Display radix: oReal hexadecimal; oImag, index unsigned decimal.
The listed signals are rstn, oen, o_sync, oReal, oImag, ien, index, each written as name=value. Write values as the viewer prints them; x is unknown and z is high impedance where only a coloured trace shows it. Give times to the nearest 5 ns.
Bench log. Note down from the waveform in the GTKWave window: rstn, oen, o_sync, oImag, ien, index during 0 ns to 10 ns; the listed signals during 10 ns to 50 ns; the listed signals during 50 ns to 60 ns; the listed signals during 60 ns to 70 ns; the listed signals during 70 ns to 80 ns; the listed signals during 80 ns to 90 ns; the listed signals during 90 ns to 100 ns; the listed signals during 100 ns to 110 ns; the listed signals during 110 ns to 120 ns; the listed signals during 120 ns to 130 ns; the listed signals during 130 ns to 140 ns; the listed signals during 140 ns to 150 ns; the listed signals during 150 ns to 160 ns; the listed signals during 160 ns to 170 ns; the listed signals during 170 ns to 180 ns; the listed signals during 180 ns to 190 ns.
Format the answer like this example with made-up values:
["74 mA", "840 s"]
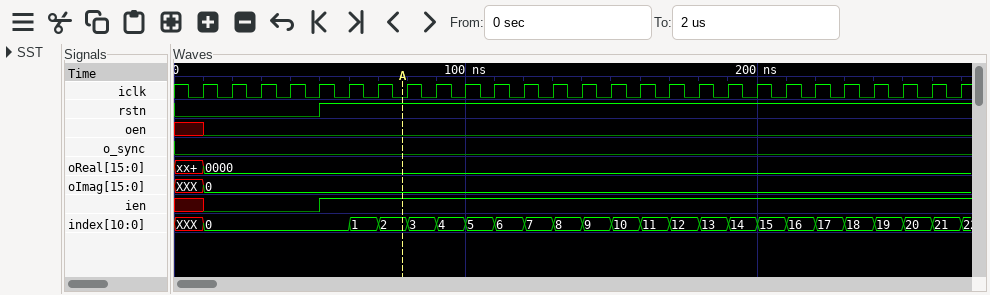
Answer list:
["rstn=0, oen=x, o_sync=0, oImag=XXX, ien=x, index=XXX", "rstn=0, oen=0, o_sync=0, oReal=0000, oImag=0, ien=0, index=0", "rstn=1, oen=0, o_sync=0, oReal=0000, oImag=0, ien=1, index=0", "rstn=1, oen=0, o_sync=0, oReal=0000, oImag=0, ien=1, index=1", "rstn=1, oen=0, o_sync=0, oReal=0000, oImag=0, ien=1, index=2", "rstn=1, oen=0, o_sync=0, oReal=0000, oImag=0, ien=1, index=3", "rstn=1, oen=0, o_sync=0, oReal=0000, oImag=0, ien=1, index=4", "rstn=1, oen=0, o_sync=0, oReal=0000, oImag=0, ien=1, index=5", "rstn=1, oen=0, o_sync=0, oReal=0000, oImag=0, ien=1, index=6", "rstn=1, oen=0, o_sync=0, oReal=0000, oImag=0, ien=1, index=7", "rstn=1, oen=0, o_sync=0, oReal=0000, oImag=0, ien=1, index=8", "rstn=1, oen=0, o_sync=0, oReal=0000, oImag=0, ien=1, index=9", "rstn=1, oen=0, o_sync=0, oReal=0000, oImag=0, ien=1, index=10", "rstn=1, oen=0, o_sync=0, oReal=0000, oImag=0, ien=1, index=11", "rstn=1, oen=0, o_sync=0, oReal=0000, oImag=0, ien=1, index=12", "rstn=1, oen=0, o_sync=0, oReal=0000, oImag=0, ien=1, index=13"]
